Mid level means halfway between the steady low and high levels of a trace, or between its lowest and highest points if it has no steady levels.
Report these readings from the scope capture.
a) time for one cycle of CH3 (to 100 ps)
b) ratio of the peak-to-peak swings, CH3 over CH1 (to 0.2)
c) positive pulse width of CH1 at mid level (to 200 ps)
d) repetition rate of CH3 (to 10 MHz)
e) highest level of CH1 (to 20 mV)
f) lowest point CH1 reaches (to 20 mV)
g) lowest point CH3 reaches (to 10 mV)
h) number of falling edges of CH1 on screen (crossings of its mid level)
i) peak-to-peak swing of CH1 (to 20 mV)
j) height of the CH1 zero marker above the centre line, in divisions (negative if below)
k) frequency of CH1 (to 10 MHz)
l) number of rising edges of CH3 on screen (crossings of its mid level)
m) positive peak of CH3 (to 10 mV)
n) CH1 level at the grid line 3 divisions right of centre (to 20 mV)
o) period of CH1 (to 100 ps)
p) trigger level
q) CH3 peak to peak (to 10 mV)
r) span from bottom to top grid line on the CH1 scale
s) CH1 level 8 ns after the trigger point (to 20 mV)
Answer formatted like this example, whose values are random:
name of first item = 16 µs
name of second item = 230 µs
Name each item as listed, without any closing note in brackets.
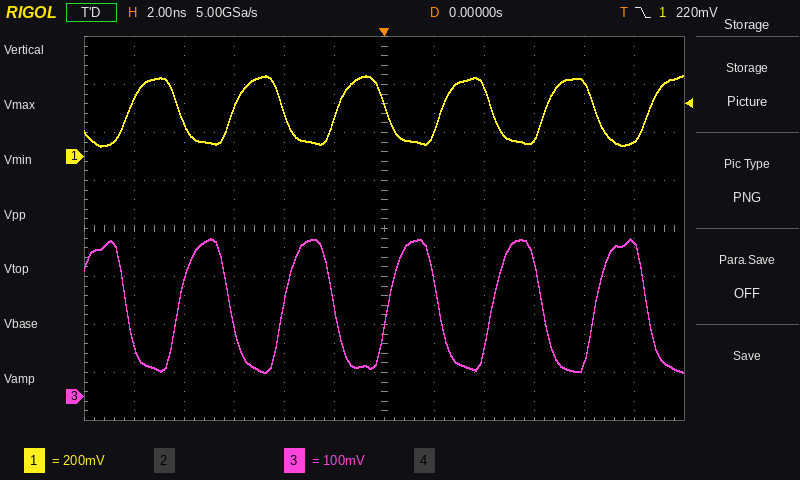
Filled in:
time for one cycle of CH3 = 4.2 ns
ratio of the peak-to-peak swings, CH3 over CH1 = 1.0
positive pulse width of CH1 at mid level = 2.0 ns
repetition rate of CH3 = 240 MHz
highest level of CH1 = 340 mV
lowest point CH1 reaches = 40 mV
lowest point CH3 reaches = 50 mV
number of falling edges of CH1 on screen = 5
peak-to-peak swing of CH1 = 300 mV
height of the CH1 zero marker above the centre line, in divisions = +1.5 div
frequency of CH1 = 240 MHz
number of rising edges of CH3 on screen = 5
positive peak of CH3 = 330 mV
CH1 level at the grid line 3 divisions right of centre = 80 mV
period of CH1 = 4.2 ns
trigger level = 220 mV
CH3 peak to peak = 280 mV
span from bottom to top grid line on the CH1 scale = 1.6 V
CH1 level 8 ns after the trigger point = 300 mV
